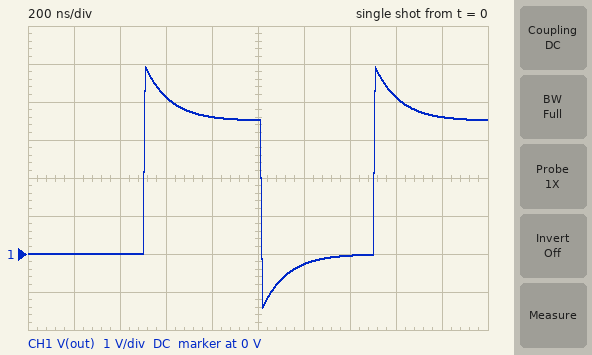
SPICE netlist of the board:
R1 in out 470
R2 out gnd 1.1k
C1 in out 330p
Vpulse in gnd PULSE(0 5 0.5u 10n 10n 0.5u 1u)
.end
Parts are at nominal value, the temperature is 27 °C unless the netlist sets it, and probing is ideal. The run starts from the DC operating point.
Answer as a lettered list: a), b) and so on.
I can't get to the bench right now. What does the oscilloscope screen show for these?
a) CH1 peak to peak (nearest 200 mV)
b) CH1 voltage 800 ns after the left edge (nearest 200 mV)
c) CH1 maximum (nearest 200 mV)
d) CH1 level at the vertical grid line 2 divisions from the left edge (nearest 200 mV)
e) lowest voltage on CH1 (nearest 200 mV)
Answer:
a) 6.4 V
b) 3.6 V
c) 5.0 V
d) 0 V
e) -1.4 V
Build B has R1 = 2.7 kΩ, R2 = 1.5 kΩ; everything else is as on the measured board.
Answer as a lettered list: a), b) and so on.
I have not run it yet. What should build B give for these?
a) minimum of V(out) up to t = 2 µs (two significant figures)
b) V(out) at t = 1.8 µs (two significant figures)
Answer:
a) -2.5 V
b) 2.8 V
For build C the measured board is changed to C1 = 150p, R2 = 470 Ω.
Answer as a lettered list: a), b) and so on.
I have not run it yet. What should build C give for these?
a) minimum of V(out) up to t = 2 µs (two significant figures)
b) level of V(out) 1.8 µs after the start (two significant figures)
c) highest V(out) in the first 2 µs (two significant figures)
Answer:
a) -2.2 V
b) 2.5 V
c) 4.7 V
